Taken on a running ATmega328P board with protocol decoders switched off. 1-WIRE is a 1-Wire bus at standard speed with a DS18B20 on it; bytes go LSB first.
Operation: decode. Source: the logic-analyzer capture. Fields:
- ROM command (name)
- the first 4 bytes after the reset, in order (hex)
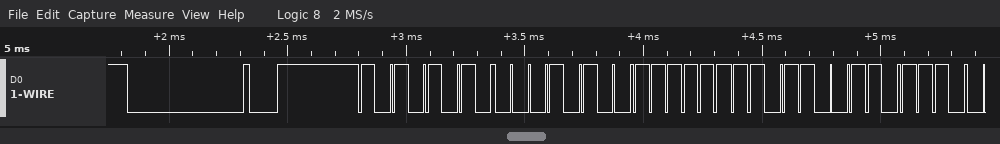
Match ROM
55 28 FF 66
